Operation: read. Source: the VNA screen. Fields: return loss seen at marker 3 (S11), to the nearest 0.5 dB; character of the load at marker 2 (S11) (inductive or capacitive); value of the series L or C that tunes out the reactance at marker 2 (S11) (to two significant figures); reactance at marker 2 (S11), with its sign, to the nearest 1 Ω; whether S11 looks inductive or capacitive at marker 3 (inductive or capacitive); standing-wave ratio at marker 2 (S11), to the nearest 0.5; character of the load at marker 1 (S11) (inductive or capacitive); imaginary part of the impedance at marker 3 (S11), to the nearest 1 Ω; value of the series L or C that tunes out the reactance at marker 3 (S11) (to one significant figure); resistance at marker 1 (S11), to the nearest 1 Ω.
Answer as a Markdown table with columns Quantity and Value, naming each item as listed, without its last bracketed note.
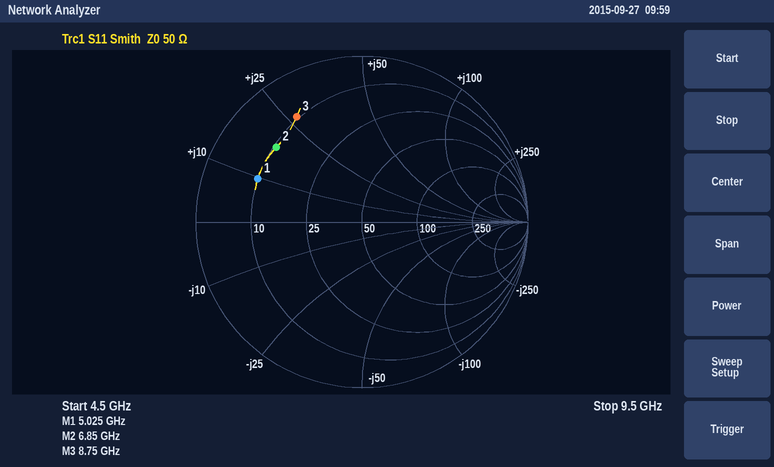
| Quantity | Value |
|---|---|
| return loss seen at marker 3 (S11), to the nearest 0.5 dB | 2.5 dB |
| character of the load at marker 2 (S11) | inductive |
| value of the series L or C that tunes out the reactance at marker 2 (S11) | 1.3 pF |
| reactance at marker 2 (S11), with its sign, to the nearest 1 Ω | +18 Ω |
| whether S11 looks inductive or capacitive at marker 3 | inductive |
| standing-wave ratio at marker 2 (S11), to the nearest 0.5 | 5.5 |
| character of the load at marker 1 (S11) | inductive |
| imaginary part of the impedance at marker 3 (S11), to the nearest 1 Ω | +27 Ω |
| value of the series L or C that tunes out the reactance at marker 3 (S11) | 700 fF |
| resistance at marker 1 (S11), to the nearest 1 Ω | 10 Ω |
